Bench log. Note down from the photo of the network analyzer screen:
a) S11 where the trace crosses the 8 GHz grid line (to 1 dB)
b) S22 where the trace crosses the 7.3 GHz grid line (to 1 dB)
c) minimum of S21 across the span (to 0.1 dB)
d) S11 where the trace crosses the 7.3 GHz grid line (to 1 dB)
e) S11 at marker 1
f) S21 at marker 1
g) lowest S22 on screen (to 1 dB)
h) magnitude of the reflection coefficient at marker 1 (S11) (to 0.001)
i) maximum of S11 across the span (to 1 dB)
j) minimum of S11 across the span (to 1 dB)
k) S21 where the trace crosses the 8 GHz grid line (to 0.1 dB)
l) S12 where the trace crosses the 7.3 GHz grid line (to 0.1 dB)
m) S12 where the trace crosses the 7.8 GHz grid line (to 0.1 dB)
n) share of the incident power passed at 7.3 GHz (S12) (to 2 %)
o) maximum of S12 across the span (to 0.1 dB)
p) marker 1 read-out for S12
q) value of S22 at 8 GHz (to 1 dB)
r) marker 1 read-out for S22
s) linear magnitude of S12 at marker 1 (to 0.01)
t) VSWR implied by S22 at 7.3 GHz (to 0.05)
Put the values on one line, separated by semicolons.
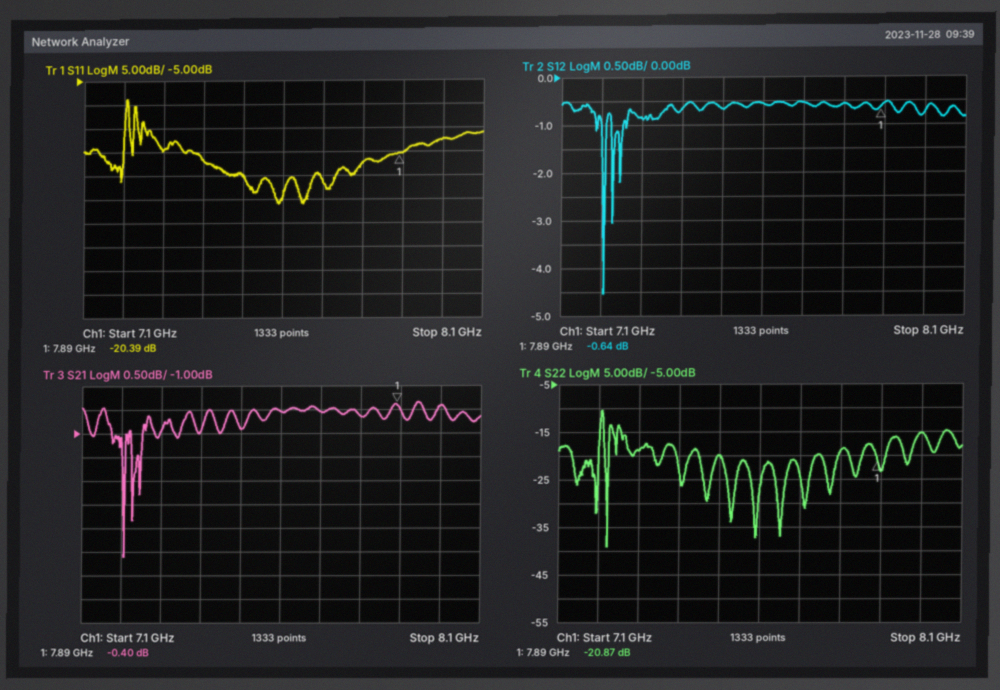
-17 dB; -19 dB; -3.6 dB; -20 dB; -20.39 dB; -0.40 dB; -39 dB; 0.096; -9 dB; -31 dB; -0.4 dB; -0.9 dB; -0.6 dB; 82 %; -0.5 dB; -0.64 dB; -15 dB; -20.87 dB; 0.93; 1.25
